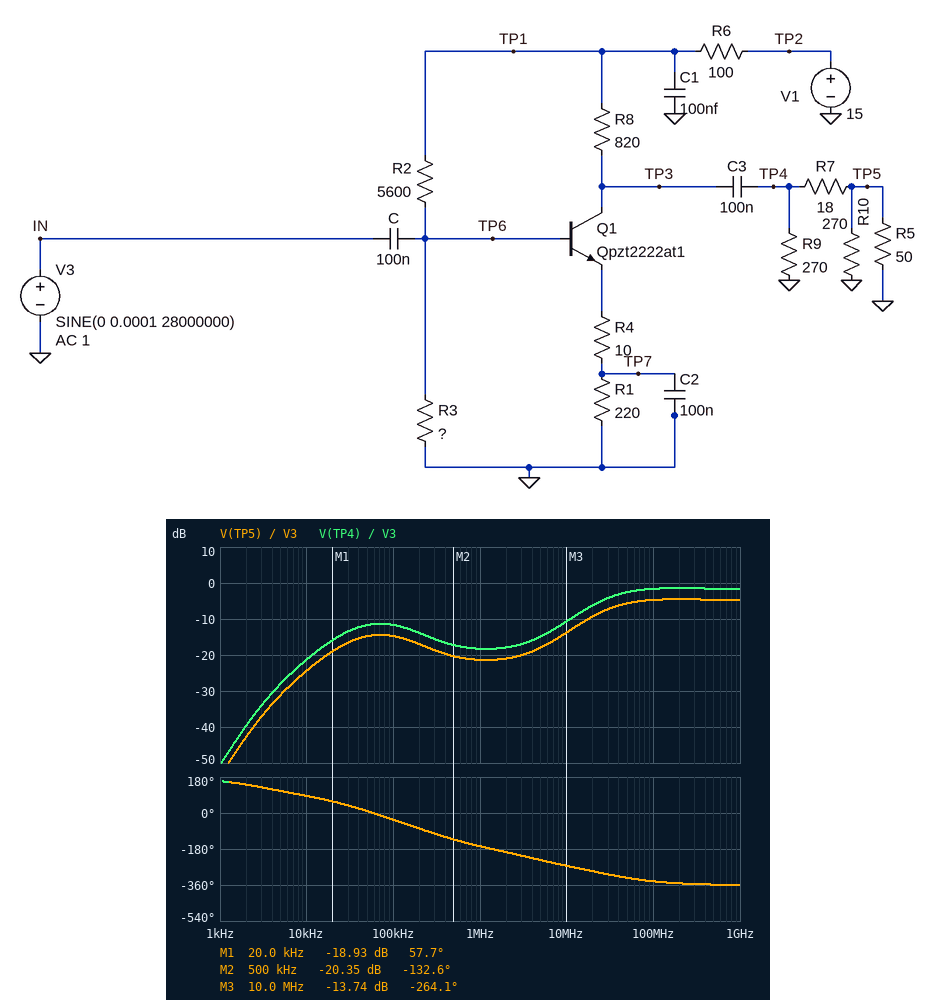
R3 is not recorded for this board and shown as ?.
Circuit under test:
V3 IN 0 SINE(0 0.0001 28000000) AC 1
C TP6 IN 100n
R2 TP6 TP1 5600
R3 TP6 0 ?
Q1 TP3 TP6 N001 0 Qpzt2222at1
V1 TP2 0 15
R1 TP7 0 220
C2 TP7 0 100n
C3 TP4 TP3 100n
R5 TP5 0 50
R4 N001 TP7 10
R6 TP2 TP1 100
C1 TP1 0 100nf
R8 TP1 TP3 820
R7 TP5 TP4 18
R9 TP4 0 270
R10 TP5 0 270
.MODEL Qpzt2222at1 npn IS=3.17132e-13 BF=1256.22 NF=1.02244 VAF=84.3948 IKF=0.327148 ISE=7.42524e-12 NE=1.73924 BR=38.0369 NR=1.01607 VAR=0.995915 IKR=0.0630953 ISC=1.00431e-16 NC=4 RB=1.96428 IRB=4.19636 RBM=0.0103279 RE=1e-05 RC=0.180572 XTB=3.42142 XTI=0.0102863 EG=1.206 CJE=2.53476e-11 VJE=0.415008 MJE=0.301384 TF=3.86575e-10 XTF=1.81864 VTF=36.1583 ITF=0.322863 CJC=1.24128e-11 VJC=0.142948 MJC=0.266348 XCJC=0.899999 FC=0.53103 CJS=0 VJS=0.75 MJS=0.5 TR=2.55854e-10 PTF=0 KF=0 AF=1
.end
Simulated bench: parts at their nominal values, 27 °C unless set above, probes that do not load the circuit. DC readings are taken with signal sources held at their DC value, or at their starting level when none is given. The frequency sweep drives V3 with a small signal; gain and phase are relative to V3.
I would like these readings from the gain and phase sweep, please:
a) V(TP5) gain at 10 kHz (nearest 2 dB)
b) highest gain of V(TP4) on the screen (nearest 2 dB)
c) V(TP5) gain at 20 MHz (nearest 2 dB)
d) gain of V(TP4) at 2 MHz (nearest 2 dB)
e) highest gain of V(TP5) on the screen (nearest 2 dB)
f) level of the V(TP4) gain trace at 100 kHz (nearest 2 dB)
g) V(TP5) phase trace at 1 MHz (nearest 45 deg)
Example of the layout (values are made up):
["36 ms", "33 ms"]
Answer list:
["-24 dB", "-2 dB", "-10 dB", "-18 dB", "-4 dB", "-12 dB", "-180 deg"]
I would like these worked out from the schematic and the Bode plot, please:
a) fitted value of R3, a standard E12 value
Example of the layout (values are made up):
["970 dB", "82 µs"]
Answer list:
["4.7 kΩ"]
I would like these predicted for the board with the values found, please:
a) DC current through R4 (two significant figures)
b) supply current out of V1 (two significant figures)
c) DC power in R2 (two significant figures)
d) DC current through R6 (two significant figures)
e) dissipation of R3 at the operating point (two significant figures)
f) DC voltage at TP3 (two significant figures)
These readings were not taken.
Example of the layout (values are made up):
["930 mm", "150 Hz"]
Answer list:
["14 mA", "14 mA", "17 mW", "14 mA", "3.1 mW", "3.2 V"]
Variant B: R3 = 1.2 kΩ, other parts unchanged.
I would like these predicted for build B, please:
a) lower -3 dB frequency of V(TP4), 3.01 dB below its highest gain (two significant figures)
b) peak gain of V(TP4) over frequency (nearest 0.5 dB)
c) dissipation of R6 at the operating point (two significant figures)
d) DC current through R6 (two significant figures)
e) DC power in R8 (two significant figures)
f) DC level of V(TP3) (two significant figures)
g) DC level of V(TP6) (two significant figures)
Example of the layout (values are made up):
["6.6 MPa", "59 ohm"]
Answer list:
["120 kHz", "10.5 dB", "9.6 mW", "9.8 mA", "49 mW", "7.7 V", "2.4 V"]
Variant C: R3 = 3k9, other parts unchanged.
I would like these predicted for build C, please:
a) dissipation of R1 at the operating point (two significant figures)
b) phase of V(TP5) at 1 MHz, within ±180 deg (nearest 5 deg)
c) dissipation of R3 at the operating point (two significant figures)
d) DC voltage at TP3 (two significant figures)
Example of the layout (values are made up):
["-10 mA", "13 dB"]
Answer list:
["40 mW", "-170 deg", "3.7 mW", "3.1 V"]
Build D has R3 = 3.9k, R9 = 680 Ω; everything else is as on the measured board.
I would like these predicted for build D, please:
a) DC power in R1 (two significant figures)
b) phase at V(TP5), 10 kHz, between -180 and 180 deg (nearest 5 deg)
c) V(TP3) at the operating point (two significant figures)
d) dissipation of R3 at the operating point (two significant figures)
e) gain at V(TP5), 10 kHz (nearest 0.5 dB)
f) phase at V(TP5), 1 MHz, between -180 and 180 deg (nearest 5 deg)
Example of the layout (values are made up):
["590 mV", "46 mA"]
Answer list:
["40 mW", "80 deg", "3.1 V", "3.7 mW", "-23.5 dB", "-170 deg"]
